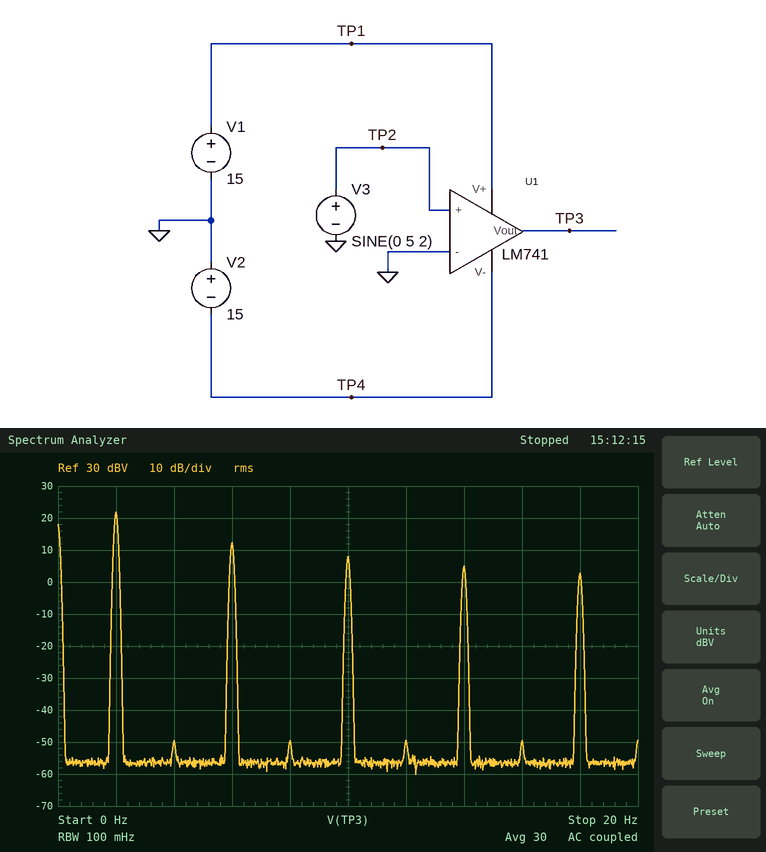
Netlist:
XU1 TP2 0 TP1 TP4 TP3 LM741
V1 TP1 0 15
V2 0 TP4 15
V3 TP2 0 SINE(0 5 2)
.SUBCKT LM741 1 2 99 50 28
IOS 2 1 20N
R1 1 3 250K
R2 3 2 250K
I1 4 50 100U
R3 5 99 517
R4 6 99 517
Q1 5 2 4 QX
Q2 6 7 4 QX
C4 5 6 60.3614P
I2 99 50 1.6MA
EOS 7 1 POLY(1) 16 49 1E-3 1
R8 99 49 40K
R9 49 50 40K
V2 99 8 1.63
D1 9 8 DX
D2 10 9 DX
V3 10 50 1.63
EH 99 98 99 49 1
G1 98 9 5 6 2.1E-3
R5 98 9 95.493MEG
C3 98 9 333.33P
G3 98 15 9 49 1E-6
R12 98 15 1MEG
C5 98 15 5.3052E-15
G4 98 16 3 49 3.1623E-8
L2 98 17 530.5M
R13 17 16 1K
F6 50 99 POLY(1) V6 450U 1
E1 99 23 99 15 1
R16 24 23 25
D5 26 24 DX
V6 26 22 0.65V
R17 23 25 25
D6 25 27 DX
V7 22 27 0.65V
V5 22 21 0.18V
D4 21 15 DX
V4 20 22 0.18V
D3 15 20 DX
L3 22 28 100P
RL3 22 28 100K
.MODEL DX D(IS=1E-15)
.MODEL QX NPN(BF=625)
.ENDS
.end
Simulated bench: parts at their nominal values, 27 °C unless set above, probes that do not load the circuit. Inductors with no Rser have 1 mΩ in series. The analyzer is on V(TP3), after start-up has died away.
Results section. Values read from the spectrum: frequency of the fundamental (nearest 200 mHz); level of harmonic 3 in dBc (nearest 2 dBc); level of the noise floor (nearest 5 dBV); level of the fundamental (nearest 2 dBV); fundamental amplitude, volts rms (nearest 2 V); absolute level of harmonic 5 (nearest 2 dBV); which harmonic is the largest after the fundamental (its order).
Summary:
2.0 Hz
-10 dBc
-55 dBV
22 dBV
12 V
8 dBV
3
